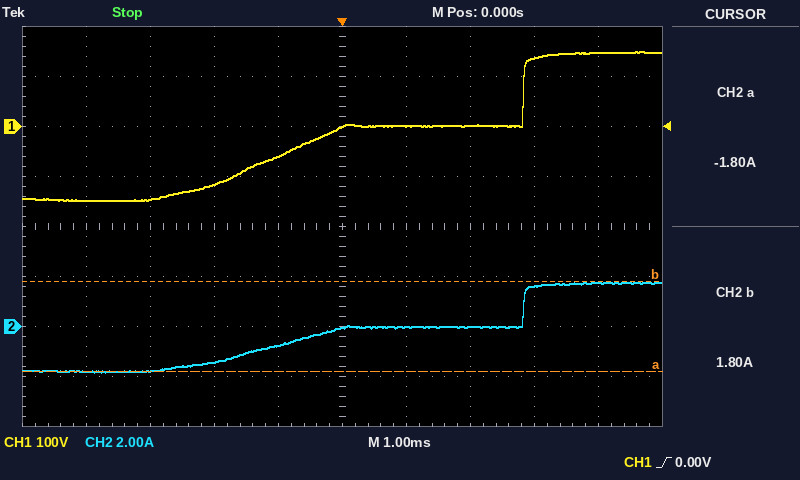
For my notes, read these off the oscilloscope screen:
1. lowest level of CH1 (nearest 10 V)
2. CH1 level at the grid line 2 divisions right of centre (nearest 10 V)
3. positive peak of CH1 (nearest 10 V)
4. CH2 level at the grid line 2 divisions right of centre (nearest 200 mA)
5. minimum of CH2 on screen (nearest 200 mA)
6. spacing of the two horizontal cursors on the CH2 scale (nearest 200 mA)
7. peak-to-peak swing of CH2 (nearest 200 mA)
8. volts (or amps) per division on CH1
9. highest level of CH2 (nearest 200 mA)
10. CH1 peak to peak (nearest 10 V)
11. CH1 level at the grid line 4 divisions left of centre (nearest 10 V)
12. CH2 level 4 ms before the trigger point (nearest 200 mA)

-150 V
0 V
150 V
0.0 A
-1.8 A
3.6 A
3.6 A
100 V
1.8 A
300 V
-150 V
-1.8 A
